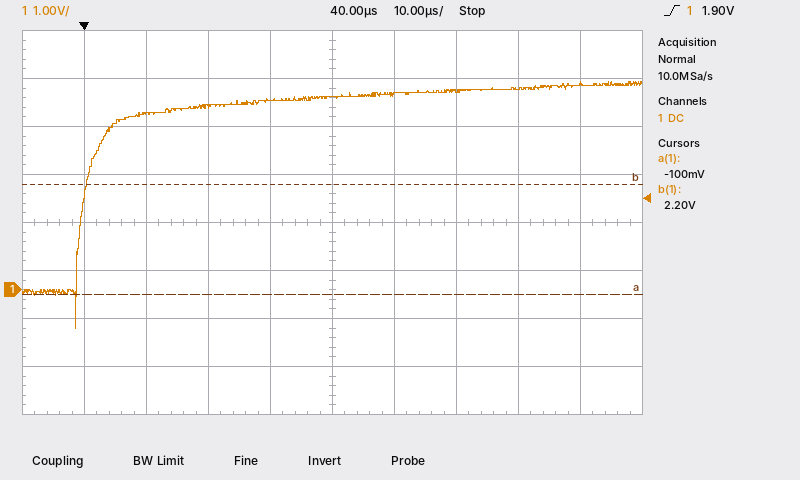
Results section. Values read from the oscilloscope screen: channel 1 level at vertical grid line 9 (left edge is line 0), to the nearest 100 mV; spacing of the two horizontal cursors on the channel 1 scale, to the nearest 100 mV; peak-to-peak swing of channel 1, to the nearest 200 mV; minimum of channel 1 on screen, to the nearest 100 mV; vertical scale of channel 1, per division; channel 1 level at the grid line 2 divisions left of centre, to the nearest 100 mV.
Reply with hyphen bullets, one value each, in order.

- 4.3 V
- 2.3 V
- 5.2 V
- -800 mV
- 1 V
- 3.8 V
